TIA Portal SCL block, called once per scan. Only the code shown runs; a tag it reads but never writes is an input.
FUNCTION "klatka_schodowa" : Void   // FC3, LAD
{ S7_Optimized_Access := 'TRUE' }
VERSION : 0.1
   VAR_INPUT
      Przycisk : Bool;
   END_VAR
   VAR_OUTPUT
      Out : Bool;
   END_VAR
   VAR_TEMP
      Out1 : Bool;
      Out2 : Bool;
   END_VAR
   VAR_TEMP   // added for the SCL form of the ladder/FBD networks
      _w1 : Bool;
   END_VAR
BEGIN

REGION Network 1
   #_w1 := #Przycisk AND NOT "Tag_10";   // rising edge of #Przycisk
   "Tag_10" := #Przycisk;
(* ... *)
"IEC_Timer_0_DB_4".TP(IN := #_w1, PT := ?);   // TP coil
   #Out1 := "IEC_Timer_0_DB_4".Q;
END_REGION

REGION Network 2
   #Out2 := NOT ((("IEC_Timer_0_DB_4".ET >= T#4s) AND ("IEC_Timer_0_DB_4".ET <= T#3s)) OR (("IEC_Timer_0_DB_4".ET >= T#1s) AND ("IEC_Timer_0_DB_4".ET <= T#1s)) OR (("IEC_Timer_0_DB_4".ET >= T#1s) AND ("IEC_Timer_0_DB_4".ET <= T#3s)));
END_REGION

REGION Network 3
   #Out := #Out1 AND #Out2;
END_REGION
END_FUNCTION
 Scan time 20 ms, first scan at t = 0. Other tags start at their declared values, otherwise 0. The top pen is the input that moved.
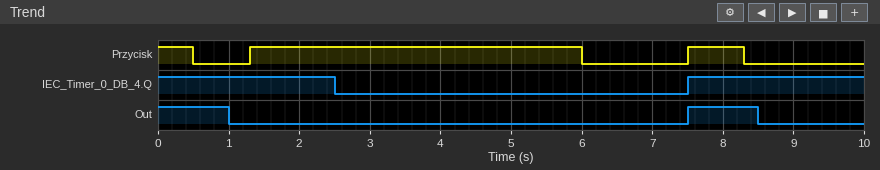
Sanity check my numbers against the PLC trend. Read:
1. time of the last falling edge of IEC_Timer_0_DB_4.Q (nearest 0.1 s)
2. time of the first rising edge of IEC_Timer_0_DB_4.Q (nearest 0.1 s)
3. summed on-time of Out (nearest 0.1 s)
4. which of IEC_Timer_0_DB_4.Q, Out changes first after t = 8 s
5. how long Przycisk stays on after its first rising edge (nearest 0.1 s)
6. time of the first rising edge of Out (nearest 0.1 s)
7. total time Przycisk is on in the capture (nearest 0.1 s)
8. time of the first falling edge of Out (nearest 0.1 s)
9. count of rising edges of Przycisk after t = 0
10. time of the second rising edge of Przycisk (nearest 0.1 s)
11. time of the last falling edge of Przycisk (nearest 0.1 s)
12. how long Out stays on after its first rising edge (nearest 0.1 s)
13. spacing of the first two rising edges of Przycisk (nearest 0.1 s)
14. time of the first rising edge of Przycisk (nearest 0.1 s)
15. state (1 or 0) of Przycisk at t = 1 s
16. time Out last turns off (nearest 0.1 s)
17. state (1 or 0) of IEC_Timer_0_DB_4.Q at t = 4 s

2.5 s
7.5 s
2.0 s
Out
4.7 s
7.5 s
6.0 s
1.0 s
2
7.5 s
8.3 s
1.0 s
6.2 s
1.3 s
0
8.5 s
0
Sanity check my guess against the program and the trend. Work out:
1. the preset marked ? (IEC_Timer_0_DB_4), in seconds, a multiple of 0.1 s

2.5 s
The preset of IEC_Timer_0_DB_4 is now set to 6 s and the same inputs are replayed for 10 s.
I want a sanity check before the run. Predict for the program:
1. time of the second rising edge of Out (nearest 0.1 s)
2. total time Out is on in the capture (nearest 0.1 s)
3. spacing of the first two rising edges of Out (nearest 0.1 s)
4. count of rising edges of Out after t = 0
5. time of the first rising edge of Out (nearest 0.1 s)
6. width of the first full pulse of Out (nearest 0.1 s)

7.5 s
5.0 s
4.5 s
2
3.0 s
3.0 s
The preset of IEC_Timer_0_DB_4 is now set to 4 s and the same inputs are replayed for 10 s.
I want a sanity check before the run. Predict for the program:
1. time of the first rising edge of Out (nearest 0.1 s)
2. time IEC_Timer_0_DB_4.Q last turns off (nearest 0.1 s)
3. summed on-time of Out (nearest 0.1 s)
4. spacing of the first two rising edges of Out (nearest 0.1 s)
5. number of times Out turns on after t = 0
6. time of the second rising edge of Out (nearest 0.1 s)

3.0 s
4.0 s
3.0 s
4.5 s
2
7.5 s
